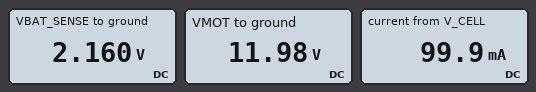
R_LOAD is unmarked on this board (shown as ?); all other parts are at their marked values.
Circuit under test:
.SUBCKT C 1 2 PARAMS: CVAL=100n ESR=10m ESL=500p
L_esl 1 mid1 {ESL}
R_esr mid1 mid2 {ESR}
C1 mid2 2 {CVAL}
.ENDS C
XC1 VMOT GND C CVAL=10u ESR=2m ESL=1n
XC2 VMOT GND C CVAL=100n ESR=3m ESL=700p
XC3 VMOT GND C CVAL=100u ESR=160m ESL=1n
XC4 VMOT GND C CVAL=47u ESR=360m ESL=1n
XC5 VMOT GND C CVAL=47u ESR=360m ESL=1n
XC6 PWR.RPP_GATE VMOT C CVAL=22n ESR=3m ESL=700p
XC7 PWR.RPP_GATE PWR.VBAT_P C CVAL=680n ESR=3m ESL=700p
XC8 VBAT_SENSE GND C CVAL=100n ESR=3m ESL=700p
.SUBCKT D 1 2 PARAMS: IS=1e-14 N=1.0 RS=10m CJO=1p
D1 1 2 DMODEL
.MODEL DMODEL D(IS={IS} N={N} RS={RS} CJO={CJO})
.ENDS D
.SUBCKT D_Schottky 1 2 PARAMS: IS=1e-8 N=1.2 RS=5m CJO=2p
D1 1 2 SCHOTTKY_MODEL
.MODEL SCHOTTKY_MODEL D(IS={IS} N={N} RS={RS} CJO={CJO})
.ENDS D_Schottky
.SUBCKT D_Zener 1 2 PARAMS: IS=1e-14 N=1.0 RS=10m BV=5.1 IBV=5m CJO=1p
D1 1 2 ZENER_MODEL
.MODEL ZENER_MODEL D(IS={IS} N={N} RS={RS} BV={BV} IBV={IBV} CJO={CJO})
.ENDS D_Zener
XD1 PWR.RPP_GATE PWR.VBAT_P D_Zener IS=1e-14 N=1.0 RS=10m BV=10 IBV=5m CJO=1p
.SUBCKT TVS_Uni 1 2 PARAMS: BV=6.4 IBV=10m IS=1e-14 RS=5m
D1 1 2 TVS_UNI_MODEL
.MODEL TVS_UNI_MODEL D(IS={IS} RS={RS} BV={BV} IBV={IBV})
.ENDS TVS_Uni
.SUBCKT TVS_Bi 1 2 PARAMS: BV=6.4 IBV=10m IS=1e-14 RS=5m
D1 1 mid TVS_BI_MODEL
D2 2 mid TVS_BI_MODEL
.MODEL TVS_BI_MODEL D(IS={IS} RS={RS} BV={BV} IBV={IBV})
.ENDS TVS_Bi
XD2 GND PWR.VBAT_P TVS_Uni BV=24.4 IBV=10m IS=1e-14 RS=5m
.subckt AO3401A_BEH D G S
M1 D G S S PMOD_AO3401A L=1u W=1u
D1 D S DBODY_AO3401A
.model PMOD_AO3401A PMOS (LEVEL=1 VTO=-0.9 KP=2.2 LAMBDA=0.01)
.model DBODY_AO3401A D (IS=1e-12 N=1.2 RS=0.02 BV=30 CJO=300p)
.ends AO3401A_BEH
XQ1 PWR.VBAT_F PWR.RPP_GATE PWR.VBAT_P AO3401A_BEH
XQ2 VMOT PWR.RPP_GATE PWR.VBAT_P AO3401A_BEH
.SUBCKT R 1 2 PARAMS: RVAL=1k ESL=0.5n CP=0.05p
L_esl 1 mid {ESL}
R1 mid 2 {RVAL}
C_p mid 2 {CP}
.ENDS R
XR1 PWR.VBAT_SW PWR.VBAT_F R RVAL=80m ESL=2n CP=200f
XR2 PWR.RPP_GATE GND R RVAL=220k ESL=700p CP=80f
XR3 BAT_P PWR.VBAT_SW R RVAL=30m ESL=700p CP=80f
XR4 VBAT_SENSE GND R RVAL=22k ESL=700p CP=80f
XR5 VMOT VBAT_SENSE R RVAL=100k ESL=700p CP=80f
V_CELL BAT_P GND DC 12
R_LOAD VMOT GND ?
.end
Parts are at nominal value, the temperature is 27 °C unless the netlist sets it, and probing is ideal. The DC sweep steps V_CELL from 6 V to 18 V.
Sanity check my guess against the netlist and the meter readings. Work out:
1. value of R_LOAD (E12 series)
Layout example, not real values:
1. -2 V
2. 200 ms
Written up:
1. 120 Ω
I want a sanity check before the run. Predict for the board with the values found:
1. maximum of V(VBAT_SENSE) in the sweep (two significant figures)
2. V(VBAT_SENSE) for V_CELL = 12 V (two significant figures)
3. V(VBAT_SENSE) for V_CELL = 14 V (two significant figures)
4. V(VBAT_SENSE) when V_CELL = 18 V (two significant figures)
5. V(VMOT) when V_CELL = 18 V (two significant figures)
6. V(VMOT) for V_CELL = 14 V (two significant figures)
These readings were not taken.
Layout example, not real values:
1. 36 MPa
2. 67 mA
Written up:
1. 3.2 V
2. 2.2 V
3. 2.5 V
4. 3.2 V
5. 18 V
6. 14 V
